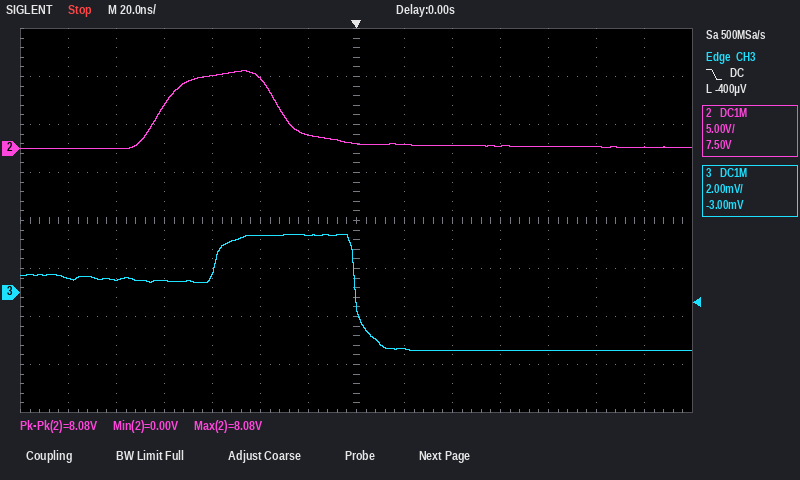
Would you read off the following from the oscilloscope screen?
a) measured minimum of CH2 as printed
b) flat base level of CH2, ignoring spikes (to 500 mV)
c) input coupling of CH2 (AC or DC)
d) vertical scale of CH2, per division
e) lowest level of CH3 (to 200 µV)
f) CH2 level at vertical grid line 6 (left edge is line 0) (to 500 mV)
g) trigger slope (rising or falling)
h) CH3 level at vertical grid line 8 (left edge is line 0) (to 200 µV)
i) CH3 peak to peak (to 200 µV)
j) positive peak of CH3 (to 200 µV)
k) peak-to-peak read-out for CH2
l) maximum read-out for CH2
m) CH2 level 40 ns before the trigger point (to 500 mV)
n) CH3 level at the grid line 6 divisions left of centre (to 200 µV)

0.00 V
0.0 V
DC
5 V
-2.4 mV
1.5 V
falling
-2.4 mV
4.8 mV
2.4 mV
8.08 V
8.08 V
7.5 V
600 µV
